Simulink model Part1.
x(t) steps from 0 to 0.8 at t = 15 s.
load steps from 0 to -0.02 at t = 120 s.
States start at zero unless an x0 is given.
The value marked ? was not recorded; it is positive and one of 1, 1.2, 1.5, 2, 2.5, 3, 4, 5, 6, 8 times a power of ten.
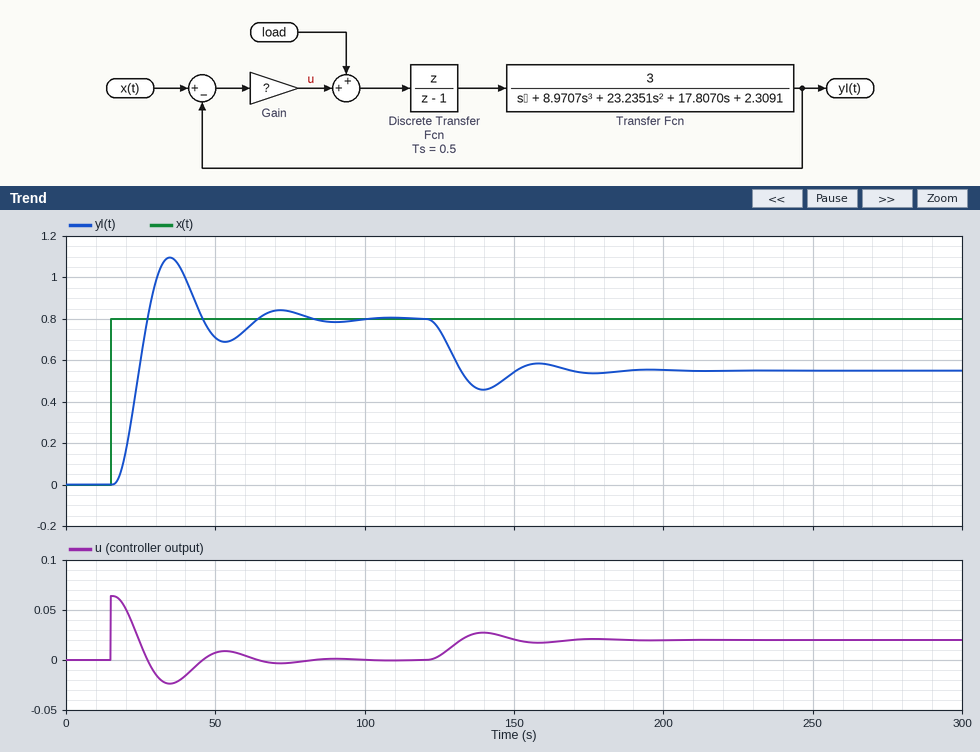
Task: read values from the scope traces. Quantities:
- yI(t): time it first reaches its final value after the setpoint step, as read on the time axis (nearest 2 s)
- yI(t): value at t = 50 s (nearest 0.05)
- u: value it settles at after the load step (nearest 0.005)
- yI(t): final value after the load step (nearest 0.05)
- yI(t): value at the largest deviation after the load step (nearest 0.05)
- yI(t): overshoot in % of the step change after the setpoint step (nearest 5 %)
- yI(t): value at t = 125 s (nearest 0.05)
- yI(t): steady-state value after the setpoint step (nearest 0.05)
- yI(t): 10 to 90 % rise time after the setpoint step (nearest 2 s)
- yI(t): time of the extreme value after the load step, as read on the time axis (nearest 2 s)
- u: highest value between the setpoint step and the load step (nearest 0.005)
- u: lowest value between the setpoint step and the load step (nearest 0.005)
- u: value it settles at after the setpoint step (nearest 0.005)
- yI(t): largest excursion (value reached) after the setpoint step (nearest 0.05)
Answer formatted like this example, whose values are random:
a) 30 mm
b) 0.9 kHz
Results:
a) 28 s
b) 0.70
c) 0.020
d) 0.55
e) 0.45
f) 35 %
g) 0.75
h) 0.80
i) 8 s
j) 140 s
k) 0.065
l) -0.025
m) 0.000
n) 1.10
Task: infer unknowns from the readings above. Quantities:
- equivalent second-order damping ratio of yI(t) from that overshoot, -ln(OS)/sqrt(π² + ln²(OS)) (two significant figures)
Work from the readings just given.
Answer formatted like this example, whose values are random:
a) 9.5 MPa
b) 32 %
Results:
a) 0.32
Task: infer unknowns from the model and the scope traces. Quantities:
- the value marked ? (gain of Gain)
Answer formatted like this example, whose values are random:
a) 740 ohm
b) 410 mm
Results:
a) 0.08
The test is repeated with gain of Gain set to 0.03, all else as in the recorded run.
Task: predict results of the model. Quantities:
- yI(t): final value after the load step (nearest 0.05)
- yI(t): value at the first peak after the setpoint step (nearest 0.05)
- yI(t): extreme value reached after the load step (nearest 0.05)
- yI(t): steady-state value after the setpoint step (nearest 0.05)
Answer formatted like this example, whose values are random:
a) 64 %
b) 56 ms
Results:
a) 0.15
b) 0.85
c) 0.10
d) 0.80
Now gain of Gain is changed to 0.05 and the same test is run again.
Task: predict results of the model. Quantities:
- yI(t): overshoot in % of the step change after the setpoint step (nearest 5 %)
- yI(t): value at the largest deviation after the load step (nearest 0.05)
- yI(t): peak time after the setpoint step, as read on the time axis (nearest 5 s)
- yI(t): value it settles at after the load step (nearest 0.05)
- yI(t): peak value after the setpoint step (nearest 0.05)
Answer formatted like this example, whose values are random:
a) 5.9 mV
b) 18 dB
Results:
a) 20 %
b) 0.30
c) 40 s
d) 0.40
e) 0.95
